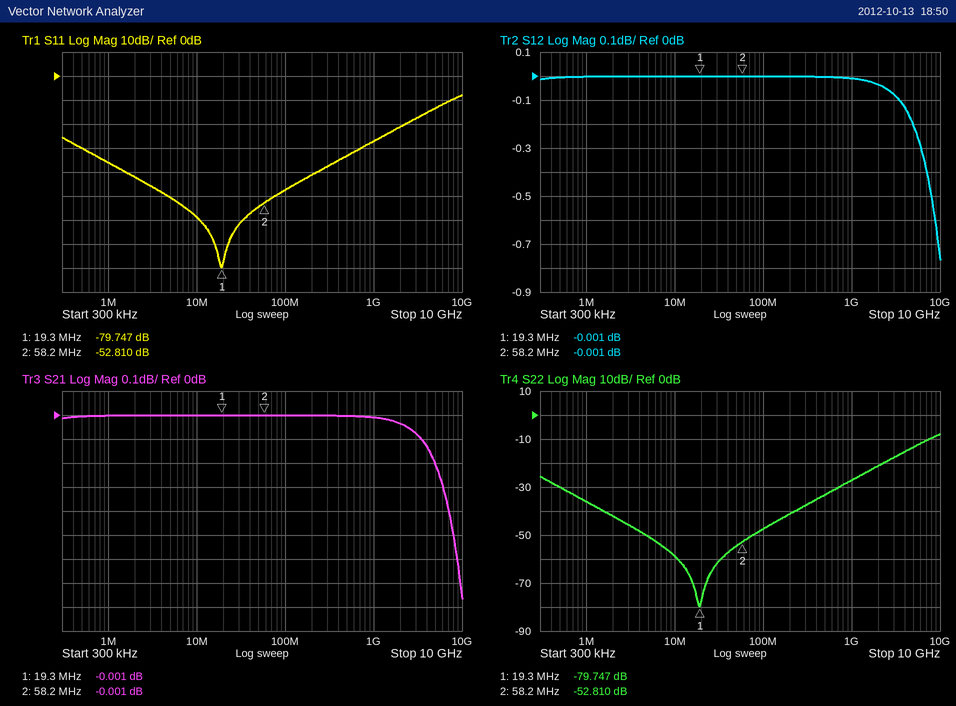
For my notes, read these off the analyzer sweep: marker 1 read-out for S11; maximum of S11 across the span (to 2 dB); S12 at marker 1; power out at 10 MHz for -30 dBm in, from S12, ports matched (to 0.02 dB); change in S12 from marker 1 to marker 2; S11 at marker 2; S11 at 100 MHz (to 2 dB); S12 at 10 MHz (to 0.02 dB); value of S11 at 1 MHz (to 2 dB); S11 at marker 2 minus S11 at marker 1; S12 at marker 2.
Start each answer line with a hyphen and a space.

- -79.747 dB
- -8 dB
- -0.001 dB
- -30.00 dBm
- 0.000 dB
- -52.810 dB
- -48 dB
- 0.00 dB
- -36 dB
- 26.937 dB
- -0.001 dB
